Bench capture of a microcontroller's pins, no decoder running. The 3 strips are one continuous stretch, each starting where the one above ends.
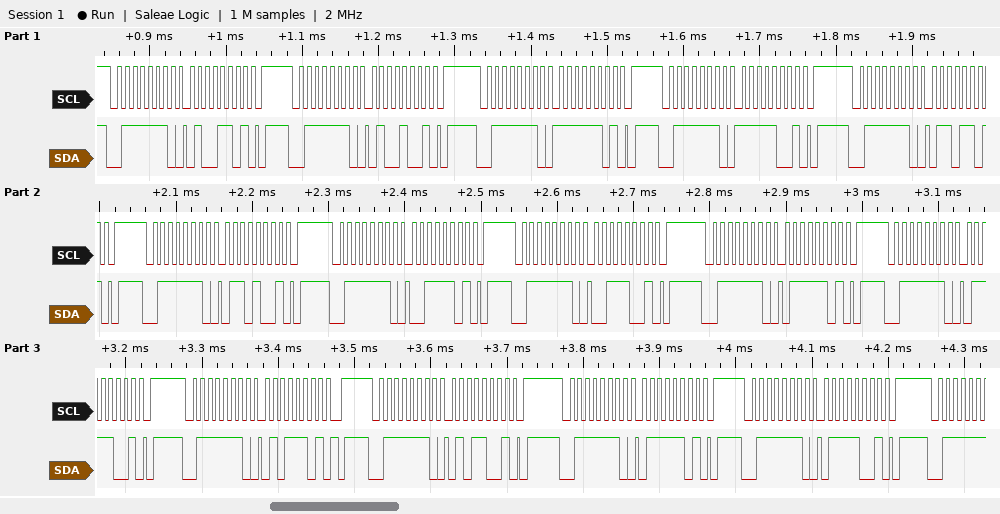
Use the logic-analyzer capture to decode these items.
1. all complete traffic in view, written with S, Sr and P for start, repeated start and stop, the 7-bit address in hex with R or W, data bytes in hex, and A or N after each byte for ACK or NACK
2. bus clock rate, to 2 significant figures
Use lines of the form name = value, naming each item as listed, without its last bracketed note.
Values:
all complete traffic in view, written with S, Sr and P for start, repeated start and stop, the 7-bit address in hex with R or W, data bytes in hex, and A or N after each byte for ACK or NACK = S 3FW A 4D A P S 3FW A 49 A P S 3FW A FD A P S 3FW A F9 A P S 3FW A 6D A P S 3FW A 69 A P S 3FW A 3D A P S 3FW A 39 A P S 3FW A 7D A P S 3FW A 79 A P S 3FW A 5D A P S 3FW A 59 A P S 3FW A 7D A P S 3FW A 79 A P
bus clock rate, to 2 significant figures = 100 kHz
